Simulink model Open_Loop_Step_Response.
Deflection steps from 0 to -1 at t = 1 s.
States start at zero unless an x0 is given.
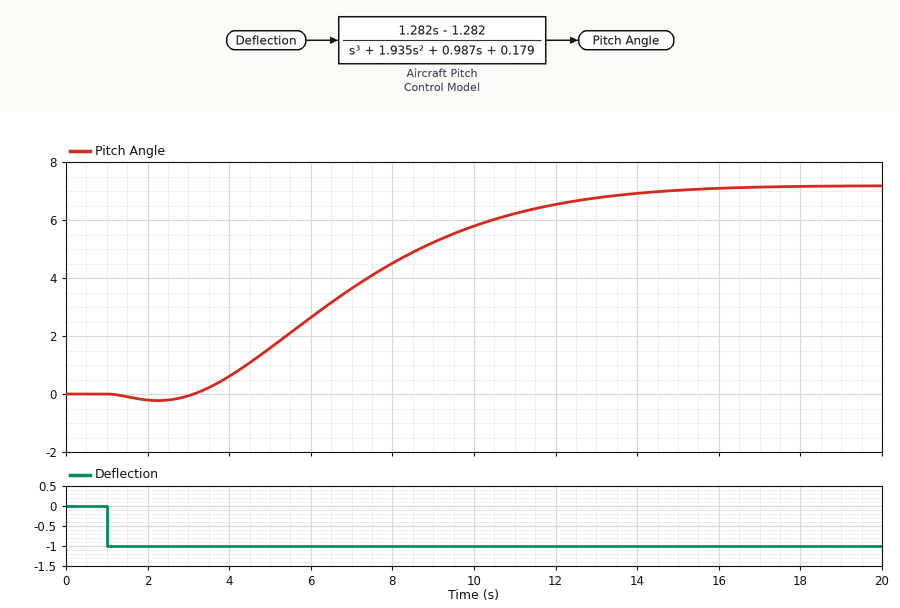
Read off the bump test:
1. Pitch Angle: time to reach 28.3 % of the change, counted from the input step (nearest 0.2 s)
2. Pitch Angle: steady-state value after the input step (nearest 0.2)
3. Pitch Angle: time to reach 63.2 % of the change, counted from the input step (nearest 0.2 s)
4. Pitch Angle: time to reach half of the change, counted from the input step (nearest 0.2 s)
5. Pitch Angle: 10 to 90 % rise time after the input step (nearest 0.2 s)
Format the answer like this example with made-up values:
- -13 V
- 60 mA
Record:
- 4.4 s
- 7.2
- 7.0 s
- 6.0 s
- 7.6 s
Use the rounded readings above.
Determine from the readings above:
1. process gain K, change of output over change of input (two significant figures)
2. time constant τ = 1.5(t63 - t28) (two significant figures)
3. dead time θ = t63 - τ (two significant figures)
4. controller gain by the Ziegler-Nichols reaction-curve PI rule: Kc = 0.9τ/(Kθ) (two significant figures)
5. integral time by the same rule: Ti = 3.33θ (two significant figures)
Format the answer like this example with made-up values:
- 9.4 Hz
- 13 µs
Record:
- -7.2
- 3.9 s
- 3.1 s
- -0.16
- 10 s
